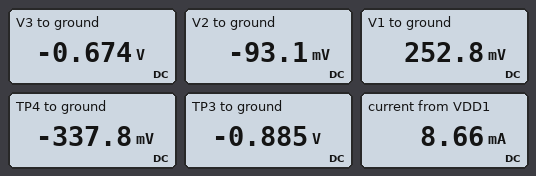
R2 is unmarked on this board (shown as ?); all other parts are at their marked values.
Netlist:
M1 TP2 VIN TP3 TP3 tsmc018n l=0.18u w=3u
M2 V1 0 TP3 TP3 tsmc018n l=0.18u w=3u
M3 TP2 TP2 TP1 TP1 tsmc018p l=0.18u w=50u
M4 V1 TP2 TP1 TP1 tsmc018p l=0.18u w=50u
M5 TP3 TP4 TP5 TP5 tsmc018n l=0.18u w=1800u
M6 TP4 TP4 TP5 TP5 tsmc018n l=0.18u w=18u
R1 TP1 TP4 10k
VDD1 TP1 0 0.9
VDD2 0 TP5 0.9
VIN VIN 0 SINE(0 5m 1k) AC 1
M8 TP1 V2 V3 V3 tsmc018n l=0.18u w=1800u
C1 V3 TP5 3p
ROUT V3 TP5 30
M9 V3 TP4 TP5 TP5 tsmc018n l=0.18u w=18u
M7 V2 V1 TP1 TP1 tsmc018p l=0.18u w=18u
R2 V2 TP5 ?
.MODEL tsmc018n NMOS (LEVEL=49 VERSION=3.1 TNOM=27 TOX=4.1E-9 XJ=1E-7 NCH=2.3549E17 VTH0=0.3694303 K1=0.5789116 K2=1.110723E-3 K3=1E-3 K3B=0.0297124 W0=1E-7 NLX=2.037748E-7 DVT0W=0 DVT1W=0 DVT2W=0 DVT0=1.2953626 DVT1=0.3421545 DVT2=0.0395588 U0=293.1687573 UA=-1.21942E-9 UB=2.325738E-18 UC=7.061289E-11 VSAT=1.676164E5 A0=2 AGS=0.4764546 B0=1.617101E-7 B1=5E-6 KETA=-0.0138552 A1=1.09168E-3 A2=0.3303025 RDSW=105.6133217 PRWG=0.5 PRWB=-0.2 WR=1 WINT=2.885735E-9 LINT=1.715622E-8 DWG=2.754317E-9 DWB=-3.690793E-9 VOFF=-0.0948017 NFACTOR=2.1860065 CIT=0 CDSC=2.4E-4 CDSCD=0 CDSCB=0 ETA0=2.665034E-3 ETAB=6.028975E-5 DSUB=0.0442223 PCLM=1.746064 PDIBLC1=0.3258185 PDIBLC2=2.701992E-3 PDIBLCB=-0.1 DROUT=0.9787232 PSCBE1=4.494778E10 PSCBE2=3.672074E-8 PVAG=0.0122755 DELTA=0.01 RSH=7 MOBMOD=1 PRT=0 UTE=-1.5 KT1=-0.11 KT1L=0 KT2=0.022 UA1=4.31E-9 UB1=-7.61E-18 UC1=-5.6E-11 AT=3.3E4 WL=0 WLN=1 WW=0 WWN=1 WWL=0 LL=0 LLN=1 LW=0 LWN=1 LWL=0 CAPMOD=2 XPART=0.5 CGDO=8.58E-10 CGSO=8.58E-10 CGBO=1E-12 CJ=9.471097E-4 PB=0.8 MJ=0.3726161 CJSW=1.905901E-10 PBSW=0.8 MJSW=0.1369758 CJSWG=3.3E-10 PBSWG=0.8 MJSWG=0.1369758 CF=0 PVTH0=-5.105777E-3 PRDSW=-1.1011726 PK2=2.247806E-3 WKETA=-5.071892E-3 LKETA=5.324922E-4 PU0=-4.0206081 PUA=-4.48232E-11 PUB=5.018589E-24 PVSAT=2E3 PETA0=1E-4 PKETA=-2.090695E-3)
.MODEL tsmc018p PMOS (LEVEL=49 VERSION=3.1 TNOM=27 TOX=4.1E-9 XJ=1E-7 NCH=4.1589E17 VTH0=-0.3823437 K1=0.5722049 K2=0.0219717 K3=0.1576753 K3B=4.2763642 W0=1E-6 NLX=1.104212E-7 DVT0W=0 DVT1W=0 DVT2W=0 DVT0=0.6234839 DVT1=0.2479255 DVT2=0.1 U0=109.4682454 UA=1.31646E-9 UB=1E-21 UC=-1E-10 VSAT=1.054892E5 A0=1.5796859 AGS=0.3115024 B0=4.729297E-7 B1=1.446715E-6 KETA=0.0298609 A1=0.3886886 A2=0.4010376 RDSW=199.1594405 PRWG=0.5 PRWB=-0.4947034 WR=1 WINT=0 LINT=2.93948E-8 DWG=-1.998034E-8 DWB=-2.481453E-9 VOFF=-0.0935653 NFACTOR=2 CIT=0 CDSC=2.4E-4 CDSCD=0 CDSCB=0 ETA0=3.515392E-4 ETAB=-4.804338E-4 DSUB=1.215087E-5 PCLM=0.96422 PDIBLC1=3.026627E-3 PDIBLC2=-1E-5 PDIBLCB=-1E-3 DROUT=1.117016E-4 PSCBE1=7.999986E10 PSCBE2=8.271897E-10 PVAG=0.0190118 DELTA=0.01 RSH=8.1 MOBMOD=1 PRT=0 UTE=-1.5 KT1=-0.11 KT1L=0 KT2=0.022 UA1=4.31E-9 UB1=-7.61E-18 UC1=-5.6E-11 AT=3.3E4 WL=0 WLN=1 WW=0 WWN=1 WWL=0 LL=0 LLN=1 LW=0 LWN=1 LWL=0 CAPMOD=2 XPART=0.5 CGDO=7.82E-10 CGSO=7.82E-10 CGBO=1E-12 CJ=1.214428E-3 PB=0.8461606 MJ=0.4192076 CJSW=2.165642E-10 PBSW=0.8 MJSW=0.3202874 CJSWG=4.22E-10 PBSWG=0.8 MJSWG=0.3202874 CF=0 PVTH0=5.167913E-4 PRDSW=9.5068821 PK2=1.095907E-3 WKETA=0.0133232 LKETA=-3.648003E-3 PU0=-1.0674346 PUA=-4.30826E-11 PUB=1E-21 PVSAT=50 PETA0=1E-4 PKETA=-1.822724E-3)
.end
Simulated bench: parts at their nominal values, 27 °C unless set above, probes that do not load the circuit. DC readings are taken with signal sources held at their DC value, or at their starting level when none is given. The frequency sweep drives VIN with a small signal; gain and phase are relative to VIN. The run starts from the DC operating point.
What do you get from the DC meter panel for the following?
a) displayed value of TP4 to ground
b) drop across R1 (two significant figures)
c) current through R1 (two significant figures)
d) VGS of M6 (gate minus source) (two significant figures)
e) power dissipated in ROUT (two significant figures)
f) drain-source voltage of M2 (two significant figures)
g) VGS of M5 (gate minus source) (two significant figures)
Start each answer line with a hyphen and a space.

- -337.8 mV
- 1.2 V
- 120 µA
- 560 mV
- 1.7 mW
- 1.1 V
- 560 mV
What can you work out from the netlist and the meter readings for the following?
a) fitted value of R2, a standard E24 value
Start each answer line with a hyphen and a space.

- 5.6 kΩ
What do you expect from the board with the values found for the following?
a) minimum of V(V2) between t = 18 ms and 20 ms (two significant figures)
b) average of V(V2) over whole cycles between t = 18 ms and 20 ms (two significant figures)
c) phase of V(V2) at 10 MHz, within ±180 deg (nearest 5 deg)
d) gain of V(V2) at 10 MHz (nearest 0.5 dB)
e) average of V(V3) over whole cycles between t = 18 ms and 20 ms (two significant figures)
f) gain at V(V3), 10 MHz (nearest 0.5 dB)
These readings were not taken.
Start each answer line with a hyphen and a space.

- -470 mV
- -66 mV
- 135 deg
- 36.5 dB
- -640 mV
- 33.0 dB
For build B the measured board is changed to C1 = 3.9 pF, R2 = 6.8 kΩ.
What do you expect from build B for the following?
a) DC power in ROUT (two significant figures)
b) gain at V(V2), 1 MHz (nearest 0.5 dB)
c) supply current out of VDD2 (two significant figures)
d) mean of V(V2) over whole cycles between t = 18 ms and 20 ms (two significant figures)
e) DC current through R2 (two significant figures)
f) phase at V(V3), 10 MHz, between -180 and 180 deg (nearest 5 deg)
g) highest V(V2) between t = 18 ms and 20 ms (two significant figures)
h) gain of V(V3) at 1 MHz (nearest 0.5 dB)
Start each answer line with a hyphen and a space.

- 3.6 mW
- 40.5 dB
- 12 mA
- 81 mV
- 140 µA
- 130 deg
- 580 mV
- 37.0 dB
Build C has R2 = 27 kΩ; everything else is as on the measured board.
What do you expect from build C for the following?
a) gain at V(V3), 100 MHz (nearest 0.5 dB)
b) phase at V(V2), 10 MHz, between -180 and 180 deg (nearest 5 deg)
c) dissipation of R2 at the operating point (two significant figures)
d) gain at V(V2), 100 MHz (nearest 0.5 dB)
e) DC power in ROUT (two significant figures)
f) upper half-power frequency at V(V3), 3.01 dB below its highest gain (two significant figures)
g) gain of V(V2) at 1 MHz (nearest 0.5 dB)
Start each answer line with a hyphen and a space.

- 5.0 dB
- 165 deg
- 110 µW
- 8.0 dB
- 25 mW
- 49 MHz
- 16.5 dB
